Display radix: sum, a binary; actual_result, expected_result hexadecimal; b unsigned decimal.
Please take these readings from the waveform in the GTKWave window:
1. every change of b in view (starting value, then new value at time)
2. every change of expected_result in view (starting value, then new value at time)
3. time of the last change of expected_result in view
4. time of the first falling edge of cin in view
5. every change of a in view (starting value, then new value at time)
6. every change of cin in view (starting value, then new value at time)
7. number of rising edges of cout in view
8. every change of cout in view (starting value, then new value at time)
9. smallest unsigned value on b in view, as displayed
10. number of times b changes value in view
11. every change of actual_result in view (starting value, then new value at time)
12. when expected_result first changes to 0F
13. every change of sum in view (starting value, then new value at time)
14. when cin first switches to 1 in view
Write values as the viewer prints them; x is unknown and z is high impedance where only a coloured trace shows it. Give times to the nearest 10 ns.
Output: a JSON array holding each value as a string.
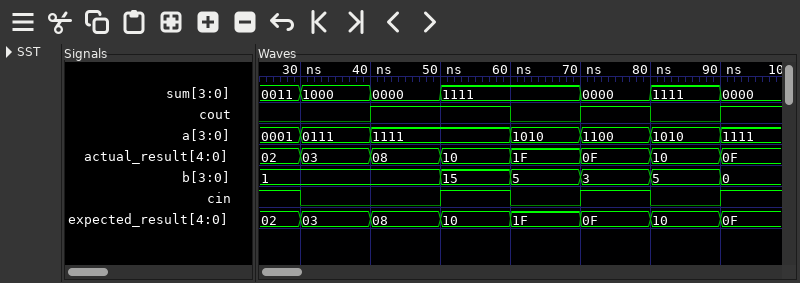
["1, 15 at 50 ns, 5 at 60 ns, 3 at 70 ns, 5 at 80 ns, 0 at 90 ns", "02, 03 at 30 ns, 08 at 40 ns, 10 at 50 ns, 1F at 60 ns, 0F at 70 ns, 10 at 80 ns, 0F at 90 ns", "90 ns", "30 ns", "0001, 0111 at 30 ns, 1111 at 40 ns, 1010 at 60 ns, 1100 at 70 ns, 1010 at 80 ns, 1111 at 90 ns", "1, 0 at 30 ns, 1 at 50 ns, 0 at 60 ns, 1 at 70 ns, 0 at 80 ns, 1 at 90 ns", "3", "0, 1 at 40 ns, 0 at 60 ns, 1 at 70 ns, 0 at 80 ns, 1 at 90 ns", "0", "5", "02, 03 at 30 ns, 08 at 40 ns, 10 at 50 ns, 1F at 60 ns, 0F at 70 ns, 10 at 80 ns, 0F at 90 ns", "70 ns", "0011, 1000 at 30 ns, 0000 at 40 ns, 1111 at 50 ns, 0000 at 70 ns, 1111 at 80 ns, 0000 at 90 ns", "50 ns"]
